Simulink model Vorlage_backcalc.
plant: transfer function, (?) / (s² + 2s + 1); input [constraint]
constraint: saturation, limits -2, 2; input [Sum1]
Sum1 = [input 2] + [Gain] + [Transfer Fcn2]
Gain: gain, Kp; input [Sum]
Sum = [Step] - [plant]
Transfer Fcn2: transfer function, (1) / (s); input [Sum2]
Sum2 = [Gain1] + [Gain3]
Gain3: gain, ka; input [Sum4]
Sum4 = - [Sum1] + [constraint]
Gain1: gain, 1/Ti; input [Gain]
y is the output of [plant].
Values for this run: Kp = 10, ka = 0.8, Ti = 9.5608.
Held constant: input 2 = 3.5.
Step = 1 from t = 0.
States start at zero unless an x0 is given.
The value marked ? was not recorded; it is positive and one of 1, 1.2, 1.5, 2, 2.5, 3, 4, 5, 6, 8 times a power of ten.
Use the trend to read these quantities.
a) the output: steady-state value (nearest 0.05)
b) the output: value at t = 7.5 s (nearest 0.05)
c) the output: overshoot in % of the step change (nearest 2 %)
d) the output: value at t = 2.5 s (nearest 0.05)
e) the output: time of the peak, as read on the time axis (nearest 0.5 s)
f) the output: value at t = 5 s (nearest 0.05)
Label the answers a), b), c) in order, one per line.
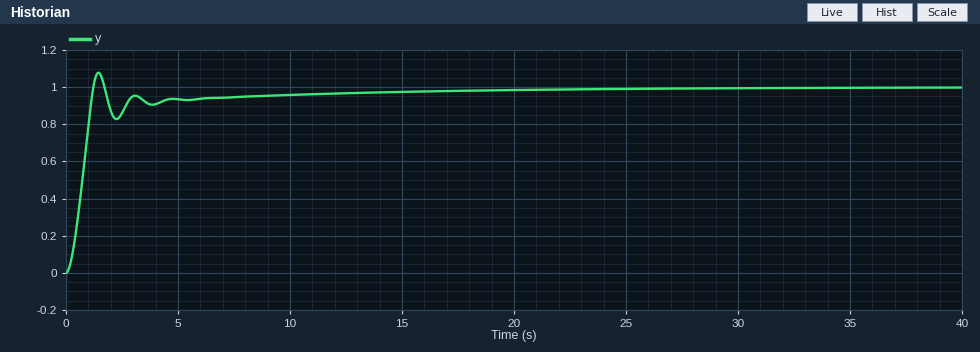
a) 1.00
b) 0.95
c) 8 %
d) 0.85
e) 1.5 s
f) 0.95
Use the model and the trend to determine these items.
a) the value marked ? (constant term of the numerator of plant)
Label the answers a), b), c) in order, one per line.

a) 1.5
